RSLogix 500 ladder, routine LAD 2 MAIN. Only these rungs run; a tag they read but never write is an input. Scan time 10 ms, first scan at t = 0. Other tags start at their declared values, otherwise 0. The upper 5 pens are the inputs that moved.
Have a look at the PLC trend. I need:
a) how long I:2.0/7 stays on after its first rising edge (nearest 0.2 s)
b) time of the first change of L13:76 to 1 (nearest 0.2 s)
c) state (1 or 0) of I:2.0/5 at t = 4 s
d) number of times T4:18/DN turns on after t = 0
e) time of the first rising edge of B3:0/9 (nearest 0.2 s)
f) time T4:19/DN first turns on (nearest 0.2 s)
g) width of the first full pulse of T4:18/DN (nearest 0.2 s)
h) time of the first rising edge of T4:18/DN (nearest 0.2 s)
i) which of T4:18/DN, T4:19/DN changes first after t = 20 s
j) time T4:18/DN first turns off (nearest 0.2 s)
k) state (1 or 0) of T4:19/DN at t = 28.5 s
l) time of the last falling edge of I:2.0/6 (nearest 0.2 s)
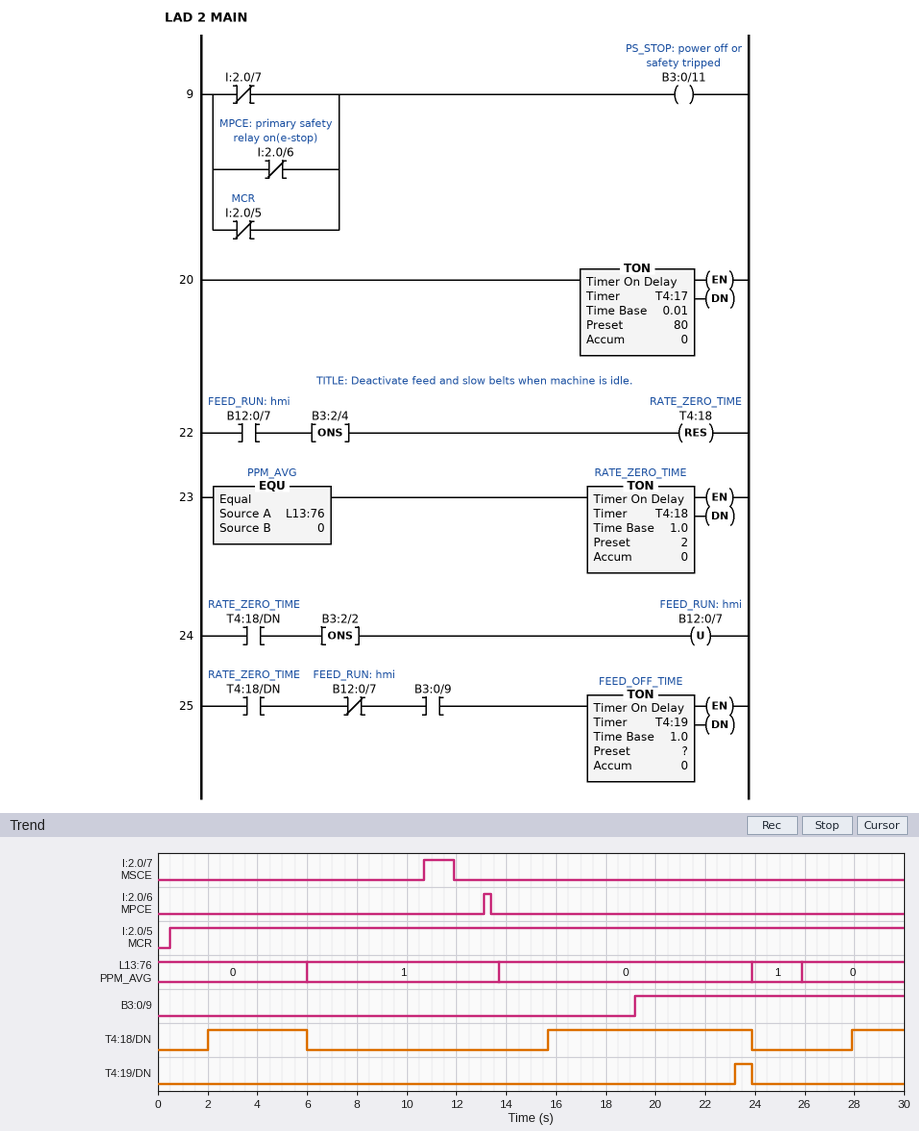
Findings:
1.2 s
6.0 s
1
3
19.2 s
23.2 s
4.0 s
2.0 s
T4:19/DN
6.0 s
0
13.4 s
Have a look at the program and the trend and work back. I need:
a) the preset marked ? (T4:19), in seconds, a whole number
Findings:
4 s
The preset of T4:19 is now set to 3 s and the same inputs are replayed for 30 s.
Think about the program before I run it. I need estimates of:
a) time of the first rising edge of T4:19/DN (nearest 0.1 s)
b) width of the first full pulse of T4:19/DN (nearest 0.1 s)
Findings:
22.2 s
1.7 s
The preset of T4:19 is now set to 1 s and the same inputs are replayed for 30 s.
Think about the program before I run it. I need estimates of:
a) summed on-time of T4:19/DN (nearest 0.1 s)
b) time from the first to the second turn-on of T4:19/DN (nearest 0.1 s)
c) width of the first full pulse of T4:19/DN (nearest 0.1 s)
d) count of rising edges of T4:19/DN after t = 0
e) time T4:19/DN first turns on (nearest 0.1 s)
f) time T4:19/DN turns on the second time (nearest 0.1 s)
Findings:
4.8 s
8.7 s
3.7 s
2
20.2 s
28.9 s
